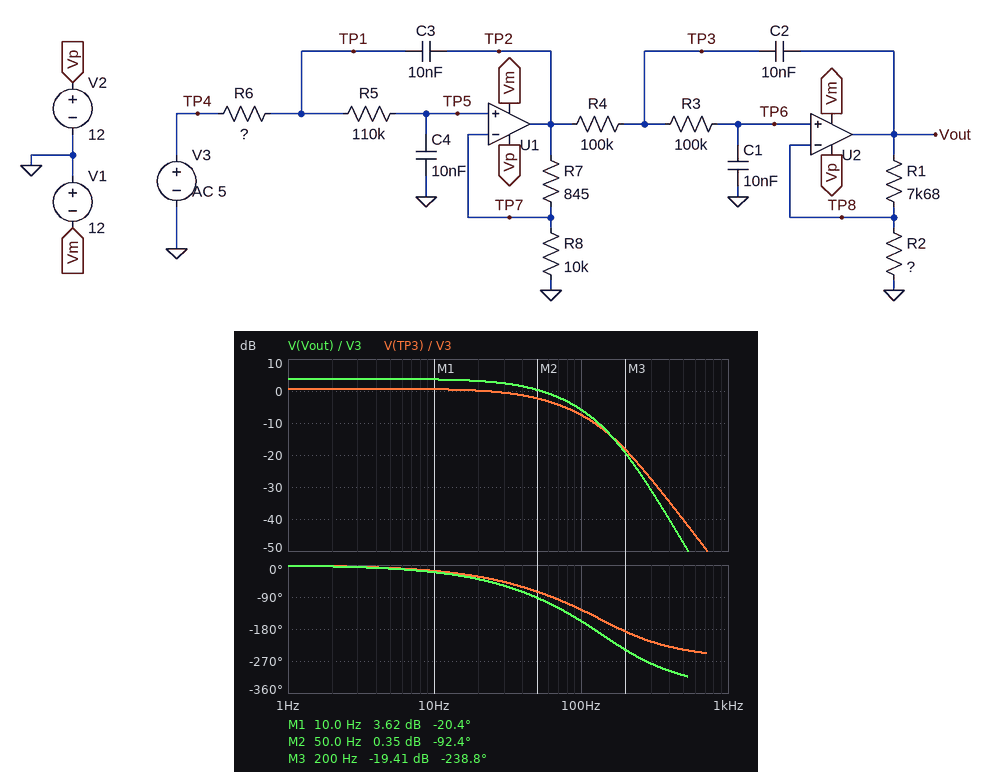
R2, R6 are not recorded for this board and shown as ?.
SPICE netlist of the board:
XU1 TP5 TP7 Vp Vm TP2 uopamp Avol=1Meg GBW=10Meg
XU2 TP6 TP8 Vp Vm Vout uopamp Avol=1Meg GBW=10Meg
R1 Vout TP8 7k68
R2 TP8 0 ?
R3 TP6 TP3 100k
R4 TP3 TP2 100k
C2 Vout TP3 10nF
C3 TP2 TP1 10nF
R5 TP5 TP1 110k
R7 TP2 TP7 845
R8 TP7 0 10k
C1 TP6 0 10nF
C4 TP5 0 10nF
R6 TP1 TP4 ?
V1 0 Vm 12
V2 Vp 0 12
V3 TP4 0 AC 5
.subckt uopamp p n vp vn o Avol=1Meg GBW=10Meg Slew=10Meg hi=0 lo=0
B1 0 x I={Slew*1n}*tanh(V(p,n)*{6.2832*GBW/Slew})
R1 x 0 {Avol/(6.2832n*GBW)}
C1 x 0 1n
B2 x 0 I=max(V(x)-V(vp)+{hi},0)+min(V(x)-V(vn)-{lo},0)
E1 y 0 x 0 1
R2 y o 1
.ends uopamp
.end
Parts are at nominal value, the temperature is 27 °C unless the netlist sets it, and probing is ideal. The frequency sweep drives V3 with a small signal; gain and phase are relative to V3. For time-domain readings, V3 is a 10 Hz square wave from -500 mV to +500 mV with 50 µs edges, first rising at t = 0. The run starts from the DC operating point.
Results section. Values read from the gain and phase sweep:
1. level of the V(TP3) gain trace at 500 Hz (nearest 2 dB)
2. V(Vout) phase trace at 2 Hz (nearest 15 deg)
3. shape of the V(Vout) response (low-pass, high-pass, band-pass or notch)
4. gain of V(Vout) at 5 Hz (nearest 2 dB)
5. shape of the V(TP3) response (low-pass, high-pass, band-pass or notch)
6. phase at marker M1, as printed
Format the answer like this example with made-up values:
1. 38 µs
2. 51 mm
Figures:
1. -40 dB
2. 0 deg
3. low-pass
4. 4 dB
5. low-pass
6. -20.4 deg
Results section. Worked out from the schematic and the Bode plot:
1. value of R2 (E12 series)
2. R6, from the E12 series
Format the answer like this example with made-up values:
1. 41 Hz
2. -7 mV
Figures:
1. 18 kΩ
2. 330 kΩ
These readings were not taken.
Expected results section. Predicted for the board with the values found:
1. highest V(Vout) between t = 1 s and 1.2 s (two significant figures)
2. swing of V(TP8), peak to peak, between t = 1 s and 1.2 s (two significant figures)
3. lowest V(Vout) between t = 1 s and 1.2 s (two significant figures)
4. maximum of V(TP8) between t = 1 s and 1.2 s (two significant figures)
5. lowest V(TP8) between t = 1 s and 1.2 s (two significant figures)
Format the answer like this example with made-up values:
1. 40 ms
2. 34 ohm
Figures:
1. 770 mV
2. 1.1 V
3. -770 mV
4. 540 mV
5. -540 mV
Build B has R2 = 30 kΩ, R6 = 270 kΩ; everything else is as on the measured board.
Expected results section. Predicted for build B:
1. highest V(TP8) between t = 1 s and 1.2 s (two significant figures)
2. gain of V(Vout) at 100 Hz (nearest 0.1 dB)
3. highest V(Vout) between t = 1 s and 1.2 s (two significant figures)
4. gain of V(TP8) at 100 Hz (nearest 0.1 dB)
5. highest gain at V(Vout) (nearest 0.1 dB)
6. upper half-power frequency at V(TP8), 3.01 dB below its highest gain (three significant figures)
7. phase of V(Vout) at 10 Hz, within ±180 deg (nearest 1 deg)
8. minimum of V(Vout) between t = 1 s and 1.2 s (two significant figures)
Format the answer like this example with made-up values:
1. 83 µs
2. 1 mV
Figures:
1. 540 mV
2. -6.3 dB
3. 680 mV
4. -8.3 dB
5. 2.7 dB
6. 50.9 Hz
7. -19 deg
8. -680 mV
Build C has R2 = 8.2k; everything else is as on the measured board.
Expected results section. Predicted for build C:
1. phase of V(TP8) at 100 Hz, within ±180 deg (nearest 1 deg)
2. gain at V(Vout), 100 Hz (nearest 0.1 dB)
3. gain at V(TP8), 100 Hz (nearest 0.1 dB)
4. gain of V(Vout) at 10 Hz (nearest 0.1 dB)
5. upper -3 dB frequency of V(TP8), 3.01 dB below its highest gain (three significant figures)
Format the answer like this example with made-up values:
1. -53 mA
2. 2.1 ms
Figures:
1. -147 deg
2. -1.0 dB
3. -6.8 dB
4. 6.3 dB
5. 51.8 Hz
